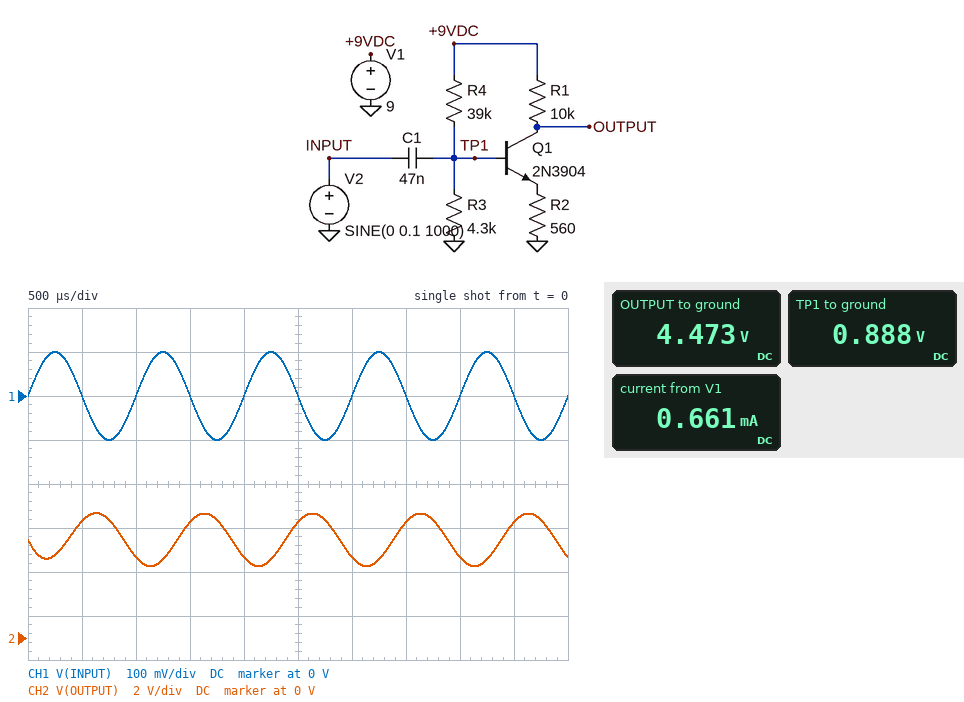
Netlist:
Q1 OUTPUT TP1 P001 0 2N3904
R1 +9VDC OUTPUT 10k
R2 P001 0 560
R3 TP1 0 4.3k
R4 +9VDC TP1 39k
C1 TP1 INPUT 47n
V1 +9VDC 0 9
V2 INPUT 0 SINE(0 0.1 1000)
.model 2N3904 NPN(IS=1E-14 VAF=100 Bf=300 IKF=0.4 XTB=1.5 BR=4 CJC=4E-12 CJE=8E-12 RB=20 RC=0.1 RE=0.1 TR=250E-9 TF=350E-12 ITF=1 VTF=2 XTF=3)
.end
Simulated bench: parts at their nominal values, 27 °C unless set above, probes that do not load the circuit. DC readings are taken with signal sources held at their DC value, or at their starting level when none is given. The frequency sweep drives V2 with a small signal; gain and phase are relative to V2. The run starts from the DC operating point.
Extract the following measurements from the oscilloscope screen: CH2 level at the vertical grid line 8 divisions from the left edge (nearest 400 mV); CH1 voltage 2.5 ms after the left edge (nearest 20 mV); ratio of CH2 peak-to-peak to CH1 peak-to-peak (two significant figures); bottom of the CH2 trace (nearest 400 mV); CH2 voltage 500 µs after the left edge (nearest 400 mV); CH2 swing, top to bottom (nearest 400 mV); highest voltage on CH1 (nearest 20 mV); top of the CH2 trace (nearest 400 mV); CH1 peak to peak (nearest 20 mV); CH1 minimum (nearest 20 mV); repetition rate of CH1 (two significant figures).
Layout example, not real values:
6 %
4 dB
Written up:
3.6 V
0 V
12
3.2 V
5.2 V
2.4 V
100 mV
5.6 V
200 mV
-100 mV
1.0 kHz
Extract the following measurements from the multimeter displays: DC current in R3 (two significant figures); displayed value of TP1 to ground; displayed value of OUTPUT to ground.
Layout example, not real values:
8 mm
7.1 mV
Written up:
210 µA
0.888 V
4.473 V
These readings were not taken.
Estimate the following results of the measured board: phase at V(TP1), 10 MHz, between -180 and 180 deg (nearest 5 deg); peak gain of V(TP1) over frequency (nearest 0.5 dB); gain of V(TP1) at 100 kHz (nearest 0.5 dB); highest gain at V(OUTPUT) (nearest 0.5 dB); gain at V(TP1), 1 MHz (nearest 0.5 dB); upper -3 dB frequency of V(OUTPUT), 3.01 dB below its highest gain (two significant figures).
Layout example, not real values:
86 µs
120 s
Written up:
0 deg
0 dB
0 dB
24.0 dB
0 dB
6.9 MHz
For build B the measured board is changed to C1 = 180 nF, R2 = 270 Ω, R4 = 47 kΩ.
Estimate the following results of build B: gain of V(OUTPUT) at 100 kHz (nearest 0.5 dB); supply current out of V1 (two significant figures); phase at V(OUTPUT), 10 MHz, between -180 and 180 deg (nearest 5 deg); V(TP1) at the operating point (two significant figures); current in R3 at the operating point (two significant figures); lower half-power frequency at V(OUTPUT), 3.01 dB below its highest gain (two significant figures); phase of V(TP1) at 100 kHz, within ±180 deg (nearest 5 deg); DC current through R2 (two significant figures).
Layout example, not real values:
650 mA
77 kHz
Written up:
29.5 dB
610 µA
120 deg
750 mV
170 µA
230 Hz
0 deg
430 µA
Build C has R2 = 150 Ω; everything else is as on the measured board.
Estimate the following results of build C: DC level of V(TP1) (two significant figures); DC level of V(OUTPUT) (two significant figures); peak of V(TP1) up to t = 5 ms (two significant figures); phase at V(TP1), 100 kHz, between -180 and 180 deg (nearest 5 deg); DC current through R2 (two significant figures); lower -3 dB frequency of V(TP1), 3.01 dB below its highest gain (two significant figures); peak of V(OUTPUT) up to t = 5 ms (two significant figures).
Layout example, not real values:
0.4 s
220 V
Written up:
790 mV
200 mV
800 mV
5 deg
910 µA
12 kHz
600 mV
